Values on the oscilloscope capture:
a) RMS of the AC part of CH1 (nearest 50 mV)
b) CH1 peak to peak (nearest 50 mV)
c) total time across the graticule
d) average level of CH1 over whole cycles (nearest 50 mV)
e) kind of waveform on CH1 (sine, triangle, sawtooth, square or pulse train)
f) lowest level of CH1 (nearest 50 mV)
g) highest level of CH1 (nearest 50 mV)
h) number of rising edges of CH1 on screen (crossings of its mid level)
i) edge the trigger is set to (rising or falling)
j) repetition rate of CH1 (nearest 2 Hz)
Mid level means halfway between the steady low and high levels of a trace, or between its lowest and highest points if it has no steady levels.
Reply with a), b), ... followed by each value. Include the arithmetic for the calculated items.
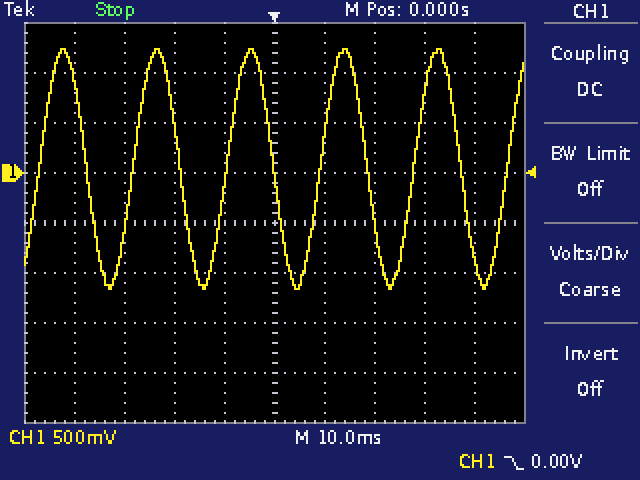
a) 2.40 V / (2√2) ≈ 849 mV, so 850 mV to the nearest 50 mV
b) 1.25 V − (-1.15 V) = 2.40 V
c) 100 ms
d) (1.25 V + (-1.15 V)) / 2 ≈ 50 mV
e) sine
f) -1.15 V
g) 1.25 V
h) 6
i) falling
j) 54 Hz
